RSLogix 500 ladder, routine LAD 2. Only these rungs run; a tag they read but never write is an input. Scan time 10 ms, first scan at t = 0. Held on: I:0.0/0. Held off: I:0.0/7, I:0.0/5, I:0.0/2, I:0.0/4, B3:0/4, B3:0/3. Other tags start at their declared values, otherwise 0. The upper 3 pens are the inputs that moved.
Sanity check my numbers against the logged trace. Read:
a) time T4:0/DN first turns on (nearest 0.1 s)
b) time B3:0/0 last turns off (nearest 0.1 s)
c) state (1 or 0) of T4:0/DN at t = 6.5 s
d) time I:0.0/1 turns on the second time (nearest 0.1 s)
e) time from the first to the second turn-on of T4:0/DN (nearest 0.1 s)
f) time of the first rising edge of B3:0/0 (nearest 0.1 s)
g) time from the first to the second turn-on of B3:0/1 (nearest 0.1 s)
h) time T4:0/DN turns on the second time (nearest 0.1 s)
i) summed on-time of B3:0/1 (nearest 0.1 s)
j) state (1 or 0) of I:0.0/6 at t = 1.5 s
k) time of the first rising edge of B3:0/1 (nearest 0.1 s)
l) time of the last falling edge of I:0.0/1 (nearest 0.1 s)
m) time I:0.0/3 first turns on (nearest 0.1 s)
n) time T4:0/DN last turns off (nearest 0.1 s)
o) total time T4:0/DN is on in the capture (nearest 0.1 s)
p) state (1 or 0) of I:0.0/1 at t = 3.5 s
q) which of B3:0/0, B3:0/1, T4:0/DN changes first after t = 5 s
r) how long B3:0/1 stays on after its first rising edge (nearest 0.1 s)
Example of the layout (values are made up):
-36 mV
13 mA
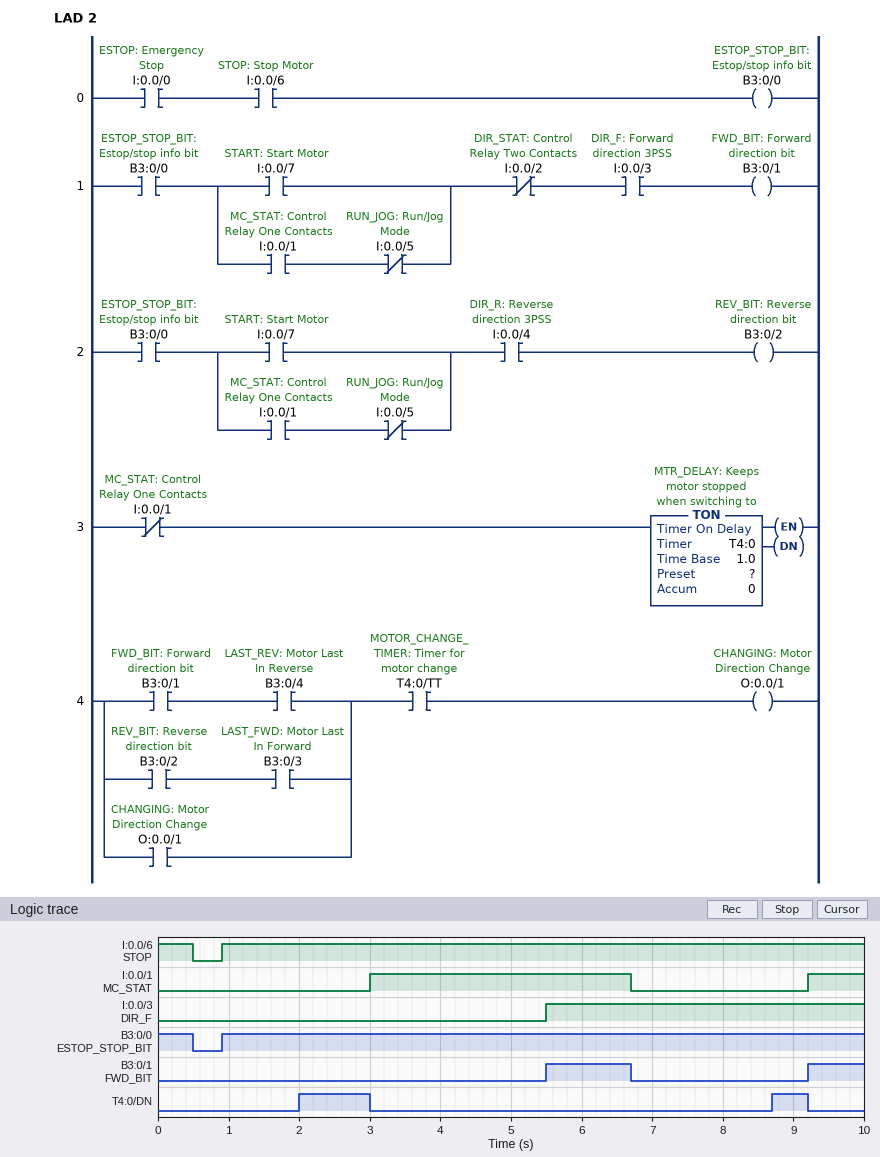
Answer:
2.0 s
0.5 s
0
9.2 s
6.7 s
0.9 s
3.7 s
8.7 s
2.0 s
1
5.5 s
6.7 s
5.5 s
9.2 s
1.5 s
1
B3:0/1
1.2 s
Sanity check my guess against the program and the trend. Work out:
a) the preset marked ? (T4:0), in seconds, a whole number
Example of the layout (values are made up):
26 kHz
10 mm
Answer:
2 s
